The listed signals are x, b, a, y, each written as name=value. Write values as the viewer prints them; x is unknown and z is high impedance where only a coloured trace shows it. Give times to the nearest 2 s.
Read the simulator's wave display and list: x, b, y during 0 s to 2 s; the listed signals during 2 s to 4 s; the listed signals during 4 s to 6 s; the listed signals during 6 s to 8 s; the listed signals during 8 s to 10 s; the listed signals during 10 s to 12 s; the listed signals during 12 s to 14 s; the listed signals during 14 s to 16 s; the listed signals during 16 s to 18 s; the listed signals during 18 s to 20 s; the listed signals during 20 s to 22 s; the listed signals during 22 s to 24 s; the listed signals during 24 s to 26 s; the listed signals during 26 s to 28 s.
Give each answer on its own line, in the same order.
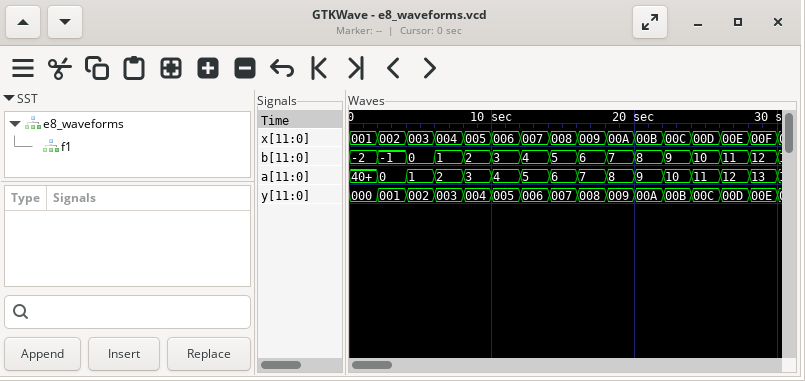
x=001, b=-2, y=000
x=002, b=-1, a=0, y=001
x=003, b=0, a=1, y=002
x=004, b=1, a=2, y=003
x=005, b=2, a=3, y=004
x=006, b=3, a=4, y=005
x=007, b=4, a=5, y=006
x=008, b=5, a=6, y=007
x=009, b=6, a=7, y=008
x=00A, b=7, a=8, y=009
x=00B, b=8, a=9, y=00A
x=00C, b=9, a=10, y=00B
x=00D, b=10, a=11, y=00C
x=00E, b=11, a=12, y=00D
